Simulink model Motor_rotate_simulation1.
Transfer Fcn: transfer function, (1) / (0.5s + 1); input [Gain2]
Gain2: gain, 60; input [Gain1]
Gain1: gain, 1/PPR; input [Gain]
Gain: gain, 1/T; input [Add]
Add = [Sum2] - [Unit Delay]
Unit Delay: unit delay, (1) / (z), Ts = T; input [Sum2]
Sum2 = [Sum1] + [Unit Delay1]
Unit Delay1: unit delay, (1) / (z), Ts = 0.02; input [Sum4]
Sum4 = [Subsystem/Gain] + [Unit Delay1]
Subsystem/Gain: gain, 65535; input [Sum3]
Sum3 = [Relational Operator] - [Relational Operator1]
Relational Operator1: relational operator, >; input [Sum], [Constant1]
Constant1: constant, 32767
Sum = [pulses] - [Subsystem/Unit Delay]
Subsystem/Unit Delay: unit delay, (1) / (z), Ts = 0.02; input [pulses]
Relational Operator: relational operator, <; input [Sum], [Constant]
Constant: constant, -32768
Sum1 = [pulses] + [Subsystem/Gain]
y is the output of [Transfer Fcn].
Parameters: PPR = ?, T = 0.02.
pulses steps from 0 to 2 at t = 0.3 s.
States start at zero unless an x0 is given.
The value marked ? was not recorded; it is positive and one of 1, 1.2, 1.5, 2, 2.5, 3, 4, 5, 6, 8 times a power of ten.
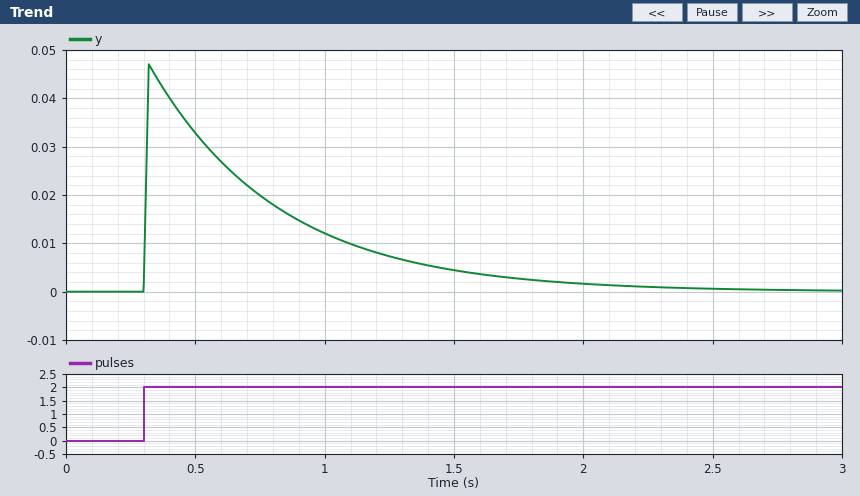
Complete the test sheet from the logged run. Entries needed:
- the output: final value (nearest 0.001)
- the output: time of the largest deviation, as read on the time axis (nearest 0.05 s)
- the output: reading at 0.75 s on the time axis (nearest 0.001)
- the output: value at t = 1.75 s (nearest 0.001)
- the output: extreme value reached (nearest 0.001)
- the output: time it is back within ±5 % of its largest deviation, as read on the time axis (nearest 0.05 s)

0.000
0.30 s
0.020
0.003
0.047
1.80 s
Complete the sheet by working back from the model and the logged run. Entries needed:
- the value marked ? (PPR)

5000
